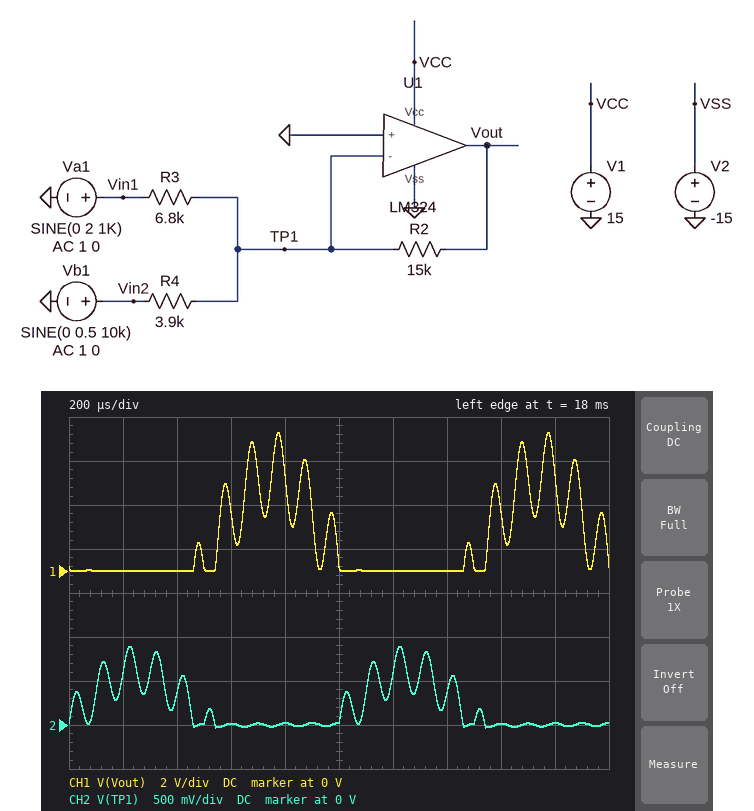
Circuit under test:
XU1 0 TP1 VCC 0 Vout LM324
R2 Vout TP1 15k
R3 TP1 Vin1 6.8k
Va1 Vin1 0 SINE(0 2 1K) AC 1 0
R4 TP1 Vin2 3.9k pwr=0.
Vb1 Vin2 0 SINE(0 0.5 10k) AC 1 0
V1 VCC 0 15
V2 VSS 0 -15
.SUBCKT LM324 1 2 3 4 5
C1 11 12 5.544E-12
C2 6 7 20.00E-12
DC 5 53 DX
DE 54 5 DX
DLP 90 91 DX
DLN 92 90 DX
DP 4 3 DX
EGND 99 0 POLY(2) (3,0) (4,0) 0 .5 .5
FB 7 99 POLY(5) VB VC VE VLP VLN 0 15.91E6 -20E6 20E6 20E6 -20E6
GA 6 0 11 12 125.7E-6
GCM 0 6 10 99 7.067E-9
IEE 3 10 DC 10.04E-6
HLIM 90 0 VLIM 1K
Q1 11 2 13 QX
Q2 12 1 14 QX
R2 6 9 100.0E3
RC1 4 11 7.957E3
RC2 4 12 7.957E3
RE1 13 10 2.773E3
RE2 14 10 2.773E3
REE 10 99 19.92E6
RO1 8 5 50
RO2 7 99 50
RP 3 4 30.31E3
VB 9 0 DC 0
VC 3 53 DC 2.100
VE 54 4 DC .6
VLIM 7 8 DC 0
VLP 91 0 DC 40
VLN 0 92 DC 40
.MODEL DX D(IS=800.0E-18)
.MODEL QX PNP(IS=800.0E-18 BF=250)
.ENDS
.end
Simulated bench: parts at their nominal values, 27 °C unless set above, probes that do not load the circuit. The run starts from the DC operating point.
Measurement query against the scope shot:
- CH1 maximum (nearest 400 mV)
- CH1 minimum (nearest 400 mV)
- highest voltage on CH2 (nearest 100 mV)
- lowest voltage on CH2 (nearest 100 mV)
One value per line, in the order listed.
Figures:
6.4 V
0 V
900 mV
0 V
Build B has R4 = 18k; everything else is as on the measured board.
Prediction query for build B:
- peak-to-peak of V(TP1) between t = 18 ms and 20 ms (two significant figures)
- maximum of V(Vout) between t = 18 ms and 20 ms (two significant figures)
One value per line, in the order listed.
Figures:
1.2 V
4.8 V
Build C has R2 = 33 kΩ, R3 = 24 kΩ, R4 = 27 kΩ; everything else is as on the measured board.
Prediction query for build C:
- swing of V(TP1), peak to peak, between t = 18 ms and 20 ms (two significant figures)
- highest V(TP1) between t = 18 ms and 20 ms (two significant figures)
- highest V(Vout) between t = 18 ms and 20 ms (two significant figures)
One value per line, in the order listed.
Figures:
940 mV
930 mV
3.3 V
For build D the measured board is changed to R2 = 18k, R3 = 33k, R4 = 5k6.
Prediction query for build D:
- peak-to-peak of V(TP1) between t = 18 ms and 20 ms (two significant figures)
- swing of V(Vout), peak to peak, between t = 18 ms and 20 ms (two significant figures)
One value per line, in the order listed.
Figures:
600 mV
2.7 V
